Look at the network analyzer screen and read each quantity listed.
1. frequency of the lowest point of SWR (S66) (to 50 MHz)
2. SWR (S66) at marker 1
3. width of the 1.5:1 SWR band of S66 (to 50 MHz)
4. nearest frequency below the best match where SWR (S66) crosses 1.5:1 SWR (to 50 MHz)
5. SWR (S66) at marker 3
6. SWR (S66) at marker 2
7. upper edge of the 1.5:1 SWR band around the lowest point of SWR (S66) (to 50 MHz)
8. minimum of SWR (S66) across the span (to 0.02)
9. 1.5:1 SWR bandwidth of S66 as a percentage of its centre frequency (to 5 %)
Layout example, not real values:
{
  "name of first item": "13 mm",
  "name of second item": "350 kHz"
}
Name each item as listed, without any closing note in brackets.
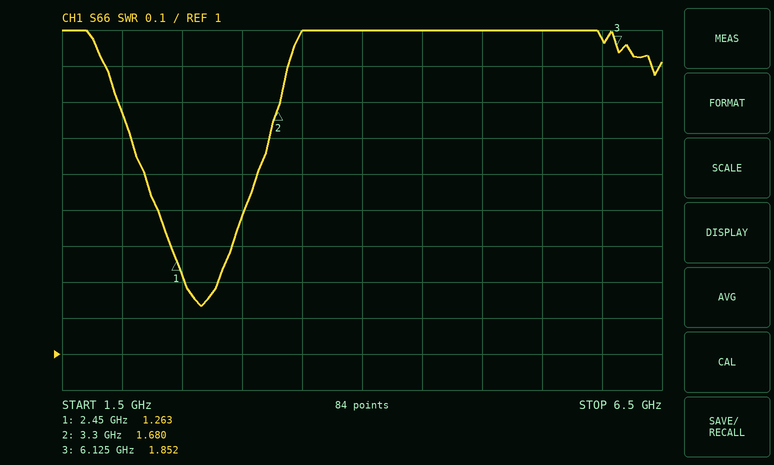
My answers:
{
  "frequency of the lowest point of SWR (S66)": "2.65 GHz",
  "SWR (S66) at marker 1": "1.263",
  "width of the 1.5:1 SWR band of S66": "950 MHz",
  "nearest frequency below the best match where SWR (S66) crosses 1.5:1 SWR": "2.20 GHz",
  "SWR (S66) at marker 3": "1.852",
  "SWR (S66) at marker 2": "1.680",
  "upper edge of the 1.5:1 SWR band around the lowest point of SWR (S66)": "3.15 GHz",
  "minimum of SWR (S66) across the span": "1.14",
  "1.5:1 SWR bandwidth of S66 as a percentage of its centre frequency": "35 %"
}
